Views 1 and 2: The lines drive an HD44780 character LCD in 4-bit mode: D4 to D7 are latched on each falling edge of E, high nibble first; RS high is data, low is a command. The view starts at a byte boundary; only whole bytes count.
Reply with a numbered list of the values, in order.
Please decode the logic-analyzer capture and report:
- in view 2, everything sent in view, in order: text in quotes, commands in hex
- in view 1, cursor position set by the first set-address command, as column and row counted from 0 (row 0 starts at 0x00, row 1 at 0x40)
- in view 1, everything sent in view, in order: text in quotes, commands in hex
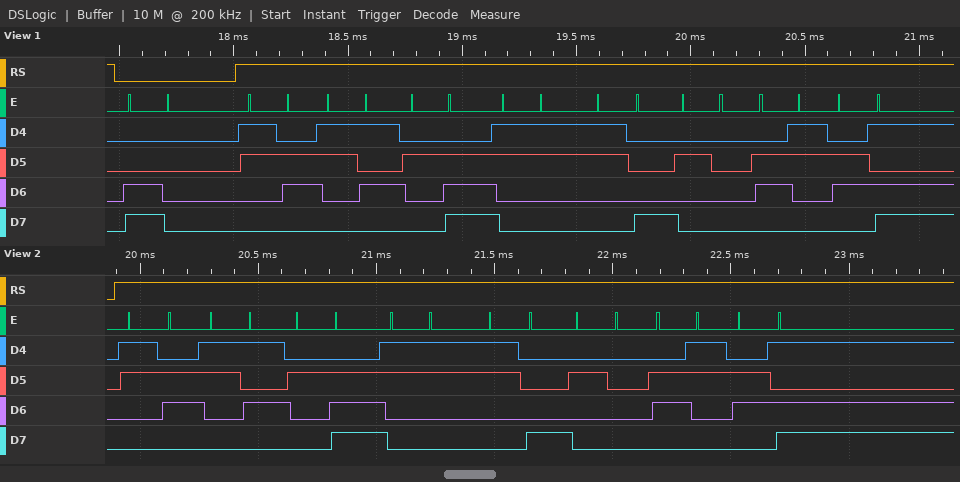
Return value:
1. "65.38 cm"
2. column 0, row 1
3. 0xC0 "65.38 cm"
